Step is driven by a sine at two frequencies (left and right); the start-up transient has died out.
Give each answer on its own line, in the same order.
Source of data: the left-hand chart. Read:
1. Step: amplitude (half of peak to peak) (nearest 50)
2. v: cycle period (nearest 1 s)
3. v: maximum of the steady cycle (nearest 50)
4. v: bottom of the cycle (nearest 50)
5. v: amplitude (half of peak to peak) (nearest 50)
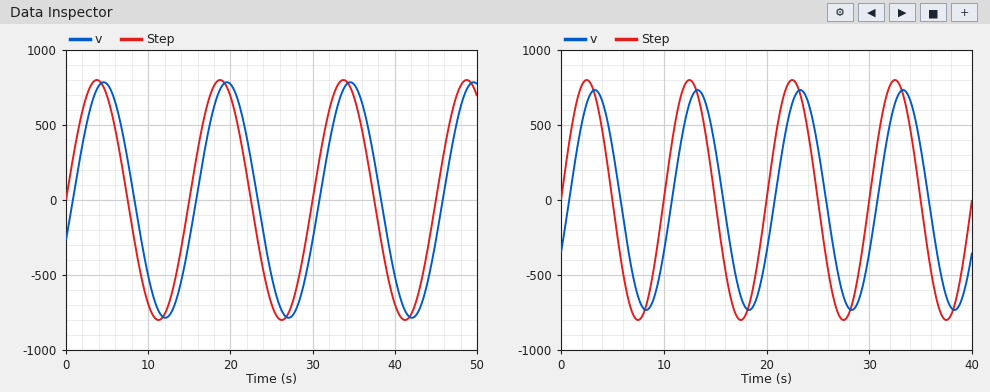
800
15 s
800
-800
800
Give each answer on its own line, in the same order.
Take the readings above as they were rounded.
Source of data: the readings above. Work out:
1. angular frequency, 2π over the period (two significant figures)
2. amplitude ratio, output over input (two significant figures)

0.42 rad/s
1.0
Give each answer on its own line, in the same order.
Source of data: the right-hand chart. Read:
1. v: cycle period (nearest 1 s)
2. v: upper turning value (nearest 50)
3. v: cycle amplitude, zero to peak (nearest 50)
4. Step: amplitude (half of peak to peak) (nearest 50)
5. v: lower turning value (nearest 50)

10 s
750
750
800
-750
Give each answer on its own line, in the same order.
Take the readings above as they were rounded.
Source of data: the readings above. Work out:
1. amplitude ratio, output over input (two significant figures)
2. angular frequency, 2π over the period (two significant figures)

0.94
0.63 rad/s
